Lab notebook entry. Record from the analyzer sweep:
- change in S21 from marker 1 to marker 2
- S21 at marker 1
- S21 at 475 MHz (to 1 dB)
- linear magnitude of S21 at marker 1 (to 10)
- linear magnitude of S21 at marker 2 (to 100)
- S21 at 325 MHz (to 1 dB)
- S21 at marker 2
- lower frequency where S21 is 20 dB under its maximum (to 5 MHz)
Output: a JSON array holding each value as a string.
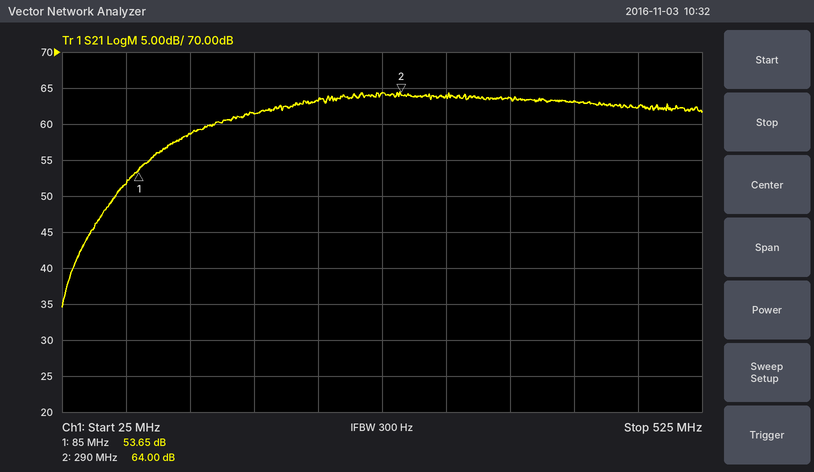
["10.35 dB", "53.65 dB", "62 dB", "480", "1600", "64 dB", "64.00 dB", "45 MHz"]
